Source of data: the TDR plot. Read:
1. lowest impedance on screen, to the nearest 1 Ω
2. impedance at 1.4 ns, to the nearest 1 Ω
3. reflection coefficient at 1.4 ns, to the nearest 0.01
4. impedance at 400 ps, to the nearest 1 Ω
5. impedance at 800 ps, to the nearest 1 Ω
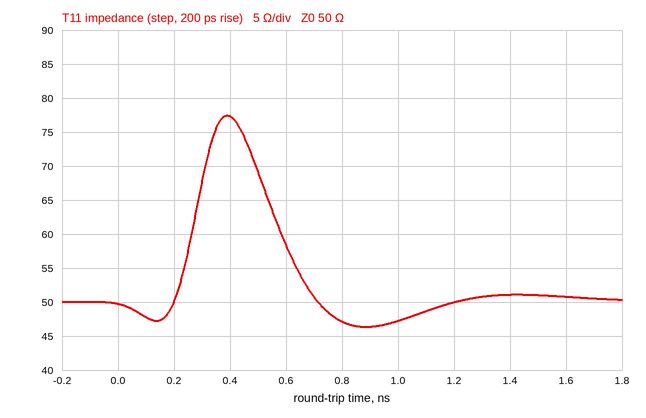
46 Ω
51 Ω
+0.01
77 Ω
47 Ω
